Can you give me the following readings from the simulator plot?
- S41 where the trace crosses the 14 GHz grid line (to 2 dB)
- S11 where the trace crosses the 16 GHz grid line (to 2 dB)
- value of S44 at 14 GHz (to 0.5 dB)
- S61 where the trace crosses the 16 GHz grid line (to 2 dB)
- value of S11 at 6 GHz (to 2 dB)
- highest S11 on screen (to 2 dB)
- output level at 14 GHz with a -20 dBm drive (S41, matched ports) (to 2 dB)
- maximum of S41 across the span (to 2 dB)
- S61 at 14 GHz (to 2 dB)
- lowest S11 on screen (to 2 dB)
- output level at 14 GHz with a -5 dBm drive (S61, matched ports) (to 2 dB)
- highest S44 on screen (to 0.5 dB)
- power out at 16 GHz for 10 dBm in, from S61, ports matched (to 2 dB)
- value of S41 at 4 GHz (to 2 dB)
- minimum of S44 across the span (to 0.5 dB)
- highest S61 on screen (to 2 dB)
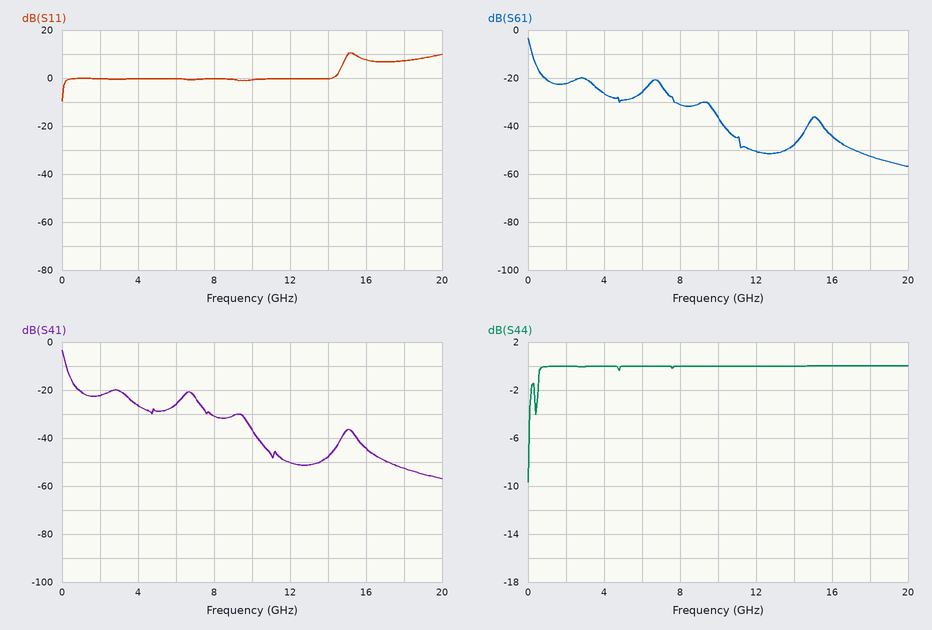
-48 dB
8 dB
0.0 dB
-44 dB
0 dB
10 dB
-68 dBm
-4 dB
-48 dB
-10 dB
-52 dBm
0.0 dB
-34 dBm
-26 dB
-9.5 dB
-4 dB
